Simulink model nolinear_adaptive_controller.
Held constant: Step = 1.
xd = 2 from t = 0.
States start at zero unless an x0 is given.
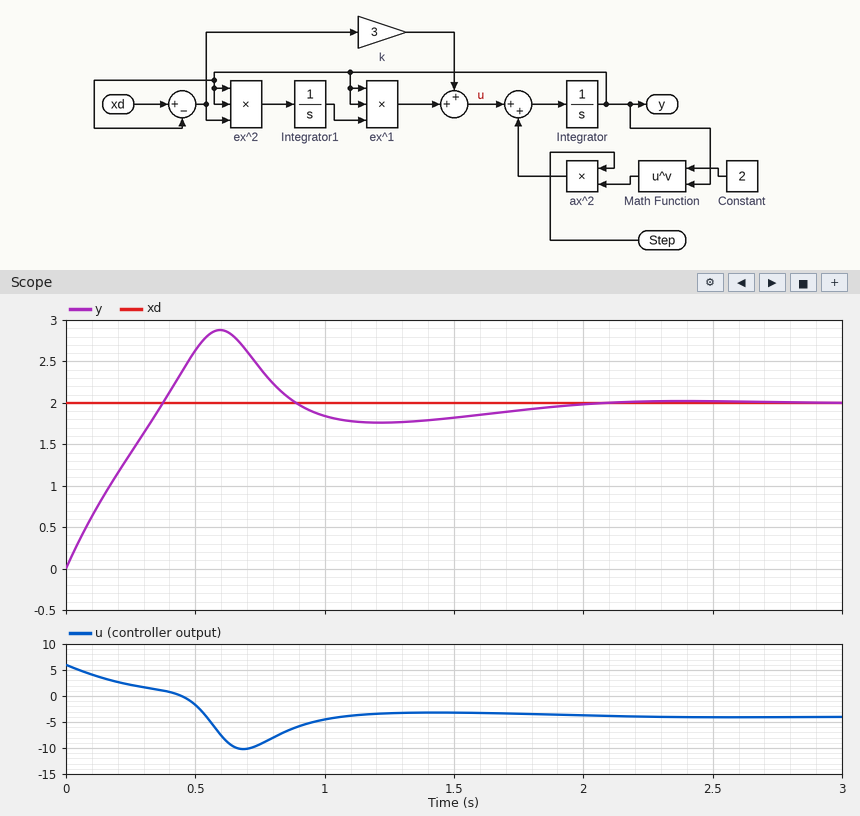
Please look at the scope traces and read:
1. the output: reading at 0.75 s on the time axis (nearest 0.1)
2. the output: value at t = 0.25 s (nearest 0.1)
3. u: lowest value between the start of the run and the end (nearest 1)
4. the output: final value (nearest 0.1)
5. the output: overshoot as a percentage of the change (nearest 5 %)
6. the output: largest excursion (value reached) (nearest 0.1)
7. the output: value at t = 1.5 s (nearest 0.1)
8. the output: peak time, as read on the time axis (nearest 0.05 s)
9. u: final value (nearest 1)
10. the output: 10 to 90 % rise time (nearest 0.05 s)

2.4
1.4
-10
2.0
45 %
2.9
1.8
0.60 s
-4
0.30 s
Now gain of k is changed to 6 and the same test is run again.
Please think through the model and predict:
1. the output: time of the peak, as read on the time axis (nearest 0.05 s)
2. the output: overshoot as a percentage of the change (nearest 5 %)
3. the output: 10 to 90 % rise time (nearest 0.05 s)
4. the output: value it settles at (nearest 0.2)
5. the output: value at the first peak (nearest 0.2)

0.50 s
30 %
0.20 s
2.0
2.6
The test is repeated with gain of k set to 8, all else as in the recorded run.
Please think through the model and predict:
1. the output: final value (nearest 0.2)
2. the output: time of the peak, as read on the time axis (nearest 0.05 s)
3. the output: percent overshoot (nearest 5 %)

2.0
0.45 s
25 %
